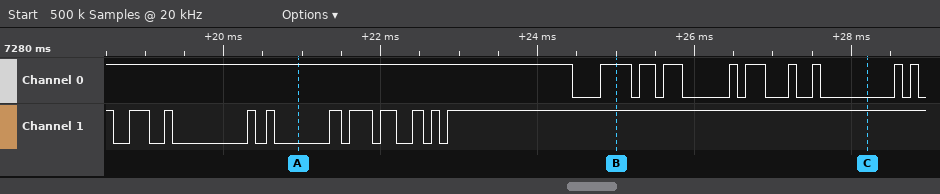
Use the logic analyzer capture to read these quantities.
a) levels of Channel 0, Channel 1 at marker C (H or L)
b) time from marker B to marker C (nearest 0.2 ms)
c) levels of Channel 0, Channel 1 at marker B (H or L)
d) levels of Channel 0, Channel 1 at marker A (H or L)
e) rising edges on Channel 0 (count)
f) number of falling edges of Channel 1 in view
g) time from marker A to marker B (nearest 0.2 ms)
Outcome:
Channel 0=L, Channel 1=H
3.2 ms
Channel 0=H, Channel 1=H
Channel 0=H, Channel 1=L
9
10
4 ms
